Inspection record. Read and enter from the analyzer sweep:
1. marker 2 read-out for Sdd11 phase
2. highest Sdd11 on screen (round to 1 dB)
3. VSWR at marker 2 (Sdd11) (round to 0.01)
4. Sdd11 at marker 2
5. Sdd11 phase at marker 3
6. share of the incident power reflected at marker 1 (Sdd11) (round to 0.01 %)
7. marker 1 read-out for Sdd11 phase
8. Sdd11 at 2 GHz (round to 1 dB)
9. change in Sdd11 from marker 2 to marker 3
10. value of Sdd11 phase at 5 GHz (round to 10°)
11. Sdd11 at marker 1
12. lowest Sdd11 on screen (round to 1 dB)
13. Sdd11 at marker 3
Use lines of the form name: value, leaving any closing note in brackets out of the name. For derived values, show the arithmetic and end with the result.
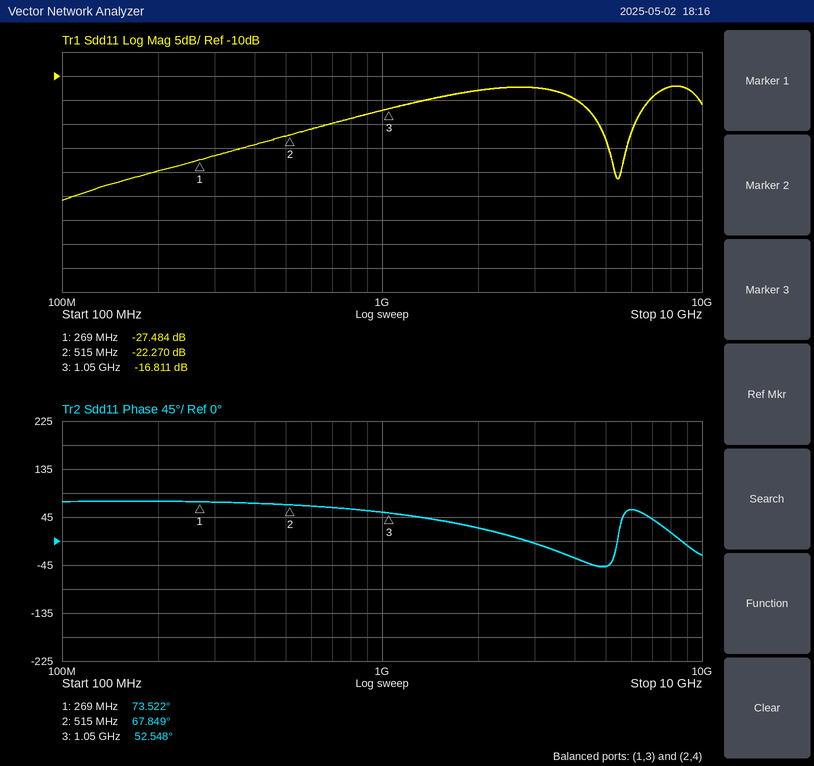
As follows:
marker 2 read-out for Sdd11 phase: 67.849°
highest Sdd11 on screen: -12 dB
VSWR at marker 2 (Sdd11): (1 + 0.0770)/(1 − 0.0770) ≈ 1.17
Sdd11 at marker 2: -22.270 dB
Sdd11 phase at marker 3: 52.548°
share of the incident power reflected at marker 1 (Sdd11): 10^(-27.484/10) ≈ 0.18 %
marker 1 read-out for Sdd11 phase: 73.522°
Sdd11 at 2 GHz: -13 dB
change in Sdd11 from marker 2 to marker 3: -16.811 − (-22.27) = 5.459 dB
value of Sdd11 phase at 5 GHz: -50°
Sdd11 at marker 1: -27.484 dB
lowest Sdd11 on screen: -36 dB
Sdd11 at marker 3: -16.811 dB
